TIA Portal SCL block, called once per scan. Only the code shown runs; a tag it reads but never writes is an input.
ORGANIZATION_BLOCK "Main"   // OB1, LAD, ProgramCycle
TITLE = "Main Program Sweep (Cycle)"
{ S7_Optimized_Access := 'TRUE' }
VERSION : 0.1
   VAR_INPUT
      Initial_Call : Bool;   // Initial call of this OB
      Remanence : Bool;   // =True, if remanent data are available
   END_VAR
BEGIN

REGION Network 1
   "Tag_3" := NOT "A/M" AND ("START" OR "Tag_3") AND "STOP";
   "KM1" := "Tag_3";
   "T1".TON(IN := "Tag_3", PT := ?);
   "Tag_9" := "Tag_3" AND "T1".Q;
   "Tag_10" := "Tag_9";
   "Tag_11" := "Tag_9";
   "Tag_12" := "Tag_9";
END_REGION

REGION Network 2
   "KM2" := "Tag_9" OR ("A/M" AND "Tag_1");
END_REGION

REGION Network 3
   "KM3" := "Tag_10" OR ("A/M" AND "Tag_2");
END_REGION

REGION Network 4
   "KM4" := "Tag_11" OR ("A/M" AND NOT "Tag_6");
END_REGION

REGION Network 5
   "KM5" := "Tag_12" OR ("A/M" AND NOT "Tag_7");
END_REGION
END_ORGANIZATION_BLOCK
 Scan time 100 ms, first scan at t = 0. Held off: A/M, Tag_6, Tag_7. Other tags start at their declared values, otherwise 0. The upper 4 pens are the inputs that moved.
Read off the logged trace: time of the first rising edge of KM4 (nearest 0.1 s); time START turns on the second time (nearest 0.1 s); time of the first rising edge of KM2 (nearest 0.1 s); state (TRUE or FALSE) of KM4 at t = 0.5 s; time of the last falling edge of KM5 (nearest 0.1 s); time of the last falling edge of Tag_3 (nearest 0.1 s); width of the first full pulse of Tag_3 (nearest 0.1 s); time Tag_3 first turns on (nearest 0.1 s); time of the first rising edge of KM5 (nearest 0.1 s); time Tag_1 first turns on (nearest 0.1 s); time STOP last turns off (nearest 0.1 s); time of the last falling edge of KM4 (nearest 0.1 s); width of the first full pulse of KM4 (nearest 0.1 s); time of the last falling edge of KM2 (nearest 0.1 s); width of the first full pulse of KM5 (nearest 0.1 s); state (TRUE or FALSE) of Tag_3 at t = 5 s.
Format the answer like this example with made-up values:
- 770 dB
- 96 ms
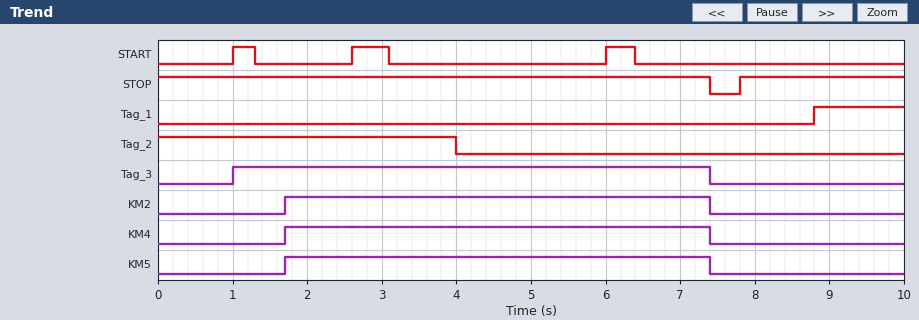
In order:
- 1.7 s
- 2.6 s
- 1.7 s
- FALSE
- 7.4 s
- 7.4 s
- 6.4 s
- 1.0 s
- 1.7 s
- 8.8 s
- 7.4 s
- 7.4 s
- 5.7 s
- 7.4 s
- 5.7 s
- TRUE
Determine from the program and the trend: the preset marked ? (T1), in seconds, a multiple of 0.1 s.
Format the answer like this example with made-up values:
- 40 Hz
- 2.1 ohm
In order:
- 0.7 s
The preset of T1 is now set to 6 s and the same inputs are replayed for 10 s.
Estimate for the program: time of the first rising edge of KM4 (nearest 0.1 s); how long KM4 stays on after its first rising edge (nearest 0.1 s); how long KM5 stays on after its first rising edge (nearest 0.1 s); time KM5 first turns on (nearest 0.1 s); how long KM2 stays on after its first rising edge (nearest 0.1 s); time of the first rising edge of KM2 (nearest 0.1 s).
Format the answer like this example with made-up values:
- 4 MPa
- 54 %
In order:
- 7.0 s
- 0.4 s
- 0.4 s
- 7.0 s
- 0.4 s
- 7.0 s
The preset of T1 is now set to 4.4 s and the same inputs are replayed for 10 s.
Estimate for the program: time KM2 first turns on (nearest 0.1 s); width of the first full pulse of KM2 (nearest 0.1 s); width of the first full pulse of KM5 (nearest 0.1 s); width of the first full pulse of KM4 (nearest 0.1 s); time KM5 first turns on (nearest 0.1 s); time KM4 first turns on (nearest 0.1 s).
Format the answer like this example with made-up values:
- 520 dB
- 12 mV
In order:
- 5.4 s
- 2.0 s
- 2.0 s
- 2.0 s
- 5.4 s
- 5.4 s
